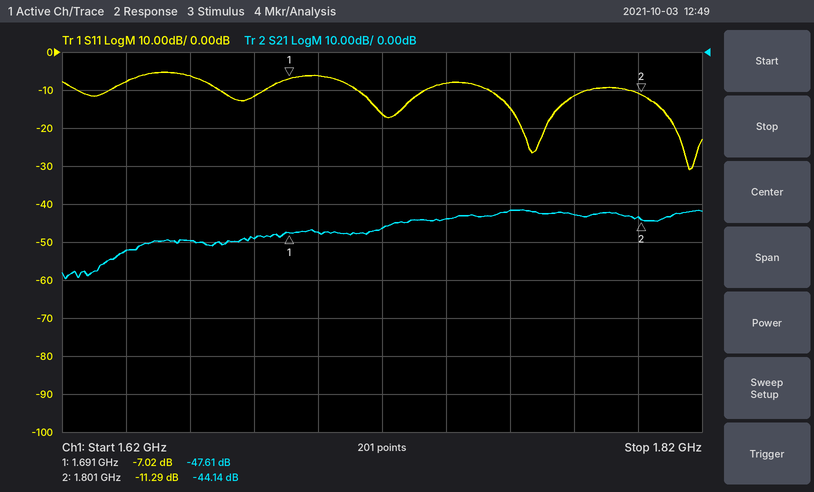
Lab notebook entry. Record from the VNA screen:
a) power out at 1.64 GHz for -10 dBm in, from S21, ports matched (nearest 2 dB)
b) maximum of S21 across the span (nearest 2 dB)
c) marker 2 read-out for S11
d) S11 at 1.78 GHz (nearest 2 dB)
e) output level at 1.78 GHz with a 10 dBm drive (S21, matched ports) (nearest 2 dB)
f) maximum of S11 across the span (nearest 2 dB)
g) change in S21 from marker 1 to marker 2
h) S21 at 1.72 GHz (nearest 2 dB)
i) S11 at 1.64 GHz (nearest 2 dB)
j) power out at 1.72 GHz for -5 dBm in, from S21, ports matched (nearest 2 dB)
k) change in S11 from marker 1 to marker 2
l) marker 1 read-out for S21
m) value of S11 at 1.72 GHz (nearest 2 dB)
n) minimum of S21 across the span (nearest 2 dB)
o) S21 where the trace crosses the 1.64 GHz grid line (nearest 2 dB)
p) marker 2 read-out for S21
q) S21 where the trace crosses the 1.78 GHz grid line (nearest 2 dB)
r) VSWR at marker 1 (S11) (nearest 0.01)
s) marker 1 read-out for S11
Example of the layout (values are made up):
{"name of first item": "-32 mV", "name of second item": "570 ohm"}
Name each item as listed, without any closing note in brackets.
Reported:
{"power out at 1.64 GHz for -10 dBm in, from S21, ports matched": "-62 dBm", "maximum of S21 across the span": "-42 dB", "marker 2 read-out for S11": "-11.29 dB", "S11 at 1.78 GHz": "-12 dB", "output level at 1.78 GHz with a 10 dBm drive (S21, matched ports)": "-32 dBm", "maximum of S11 across the span": "-6 dB", "change in S21 from marker 1 to marker 2": "3.47 dB", "S21 at 1.72 GHz": "-46 dB", "S11 at 1.64 GHz": "-8 dB", "power out at 1.72 GHz for -5 dBm in, from S21, ports matched": "-52 dBm", "change in S11 from marker 1 to marker 2": "-4.27 dB", "marker 1 read-out for S21": "-47.61 dB", "value of S11 at 1.72 GHz": "-16 dB", "minimum of S21 across the span": "-60 dB", "S21 where the trace crosses the 1.64 GHz grid line": "-52 dB", "marker 2 read-out for S21": "-44.14 dB", "S21 where the trace crosses the 1.78 GHz grid line": "-42 dB", "VSWR at marker 1 (S11)": "2.61", "marker 1 read-out for S11": "-7.02 dB"}
